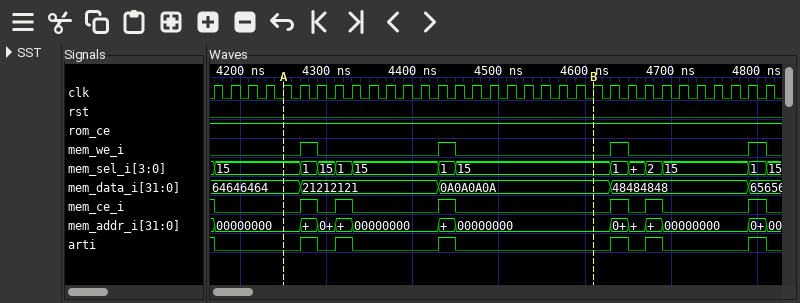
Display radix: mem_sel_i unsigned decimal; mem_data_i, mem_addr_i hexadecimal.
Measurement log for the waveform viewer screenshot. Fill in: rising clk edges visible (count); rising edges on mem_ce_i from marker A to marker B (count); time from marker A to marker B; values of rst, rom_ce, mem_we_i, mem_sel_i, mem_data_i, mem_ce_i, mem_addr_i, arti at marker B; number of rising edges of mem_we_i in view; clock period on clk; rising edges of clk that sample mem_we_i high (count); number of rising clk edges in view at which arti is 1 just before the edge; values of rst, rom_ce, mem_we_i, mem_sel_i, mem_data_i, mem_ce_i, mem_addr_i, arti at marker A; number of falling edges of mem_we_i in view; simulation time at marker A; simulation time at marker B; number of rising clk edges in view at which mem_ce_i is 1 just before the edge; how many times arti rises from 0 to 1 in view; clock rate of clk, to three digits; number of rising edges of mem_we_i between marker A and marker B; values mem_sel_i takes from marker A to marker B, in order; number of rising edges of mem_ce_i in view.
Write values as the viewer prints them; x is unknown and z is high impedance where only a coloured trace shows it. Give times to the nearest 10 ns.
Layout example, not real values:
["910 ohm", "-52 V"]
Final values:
["33", "3", "360 ns", "rst=0, rom_ce=1, mem_we_i=0, mem_sel_i=15, mem_data_i=0A0A0A0A, mem_ce_i=0, mem_addr_i=00000000, arti=0", "4", "20 ns", "4", "7", "rst=0, rom_ce=1, mem_we_i=0, mem_sel_i=15, mem_data_i=64646464, mem_ce_i=0, mem_addr_i=00000000, arti=0", "4", "4250 ns", "4610 ns", "7", "6", "50.0 MHz", "2", "15, 1, 15, 1, 15, 1, 15", "6"]
